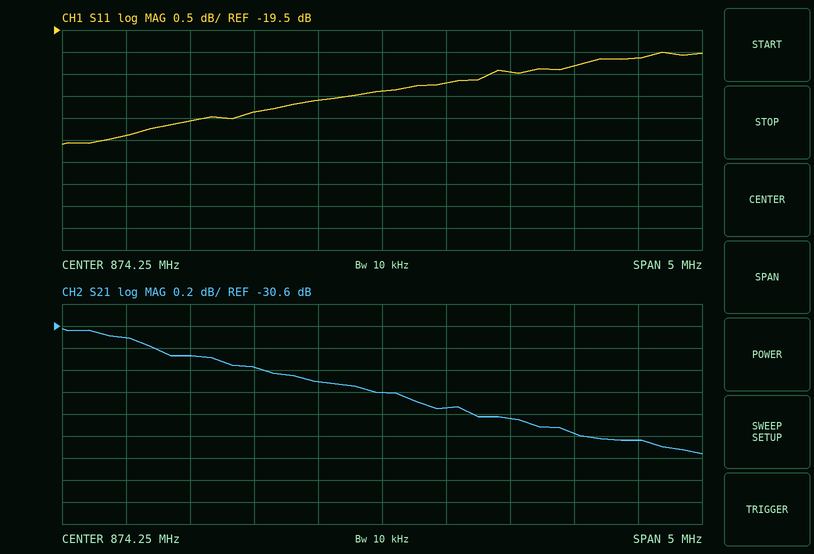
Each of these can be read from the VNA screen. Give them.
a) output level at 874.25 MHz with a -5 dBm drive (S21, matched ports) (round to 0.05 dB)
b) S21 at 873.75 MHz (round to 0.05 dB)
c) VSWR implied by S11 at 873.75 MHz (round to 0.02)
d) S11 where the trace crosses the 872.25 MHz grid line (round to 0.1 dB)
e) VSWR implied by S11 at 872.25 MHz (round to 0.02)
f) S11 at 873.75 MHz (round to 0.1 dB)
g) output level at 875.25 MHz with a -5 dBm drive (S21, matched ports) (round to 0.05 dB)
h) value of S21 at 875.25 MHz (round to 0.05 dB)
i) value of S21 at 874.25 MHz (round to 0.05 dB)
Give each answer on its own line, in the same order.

-36.20 dBm
-31.10 dB
1.20
-21.9 dB
1.18
-21.1 dB
-36.45 dBm
-31.45 dB
-31.20 dB
